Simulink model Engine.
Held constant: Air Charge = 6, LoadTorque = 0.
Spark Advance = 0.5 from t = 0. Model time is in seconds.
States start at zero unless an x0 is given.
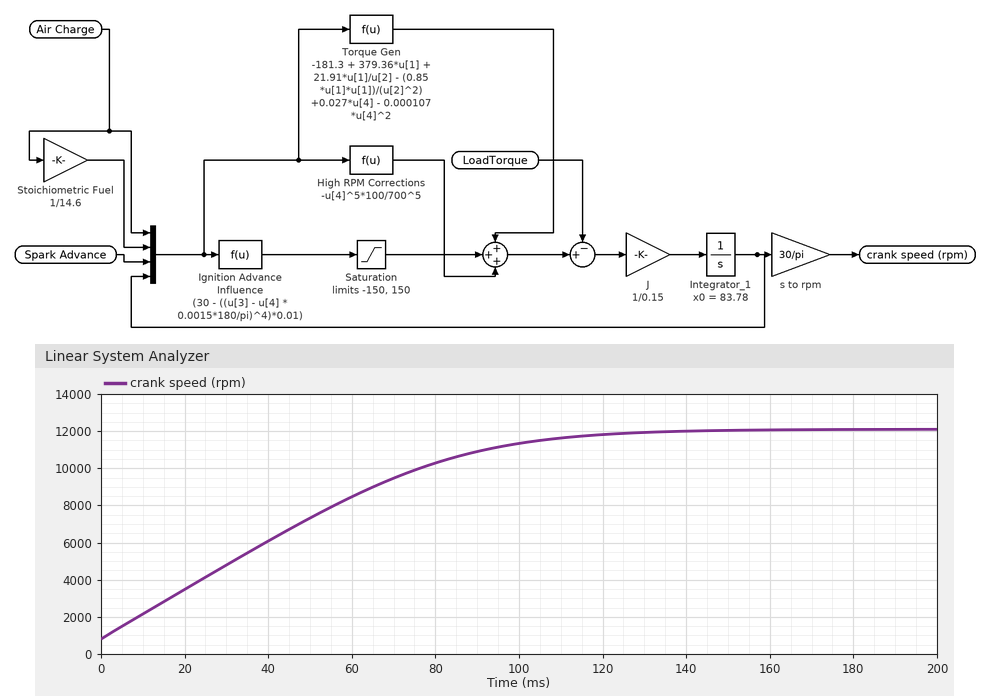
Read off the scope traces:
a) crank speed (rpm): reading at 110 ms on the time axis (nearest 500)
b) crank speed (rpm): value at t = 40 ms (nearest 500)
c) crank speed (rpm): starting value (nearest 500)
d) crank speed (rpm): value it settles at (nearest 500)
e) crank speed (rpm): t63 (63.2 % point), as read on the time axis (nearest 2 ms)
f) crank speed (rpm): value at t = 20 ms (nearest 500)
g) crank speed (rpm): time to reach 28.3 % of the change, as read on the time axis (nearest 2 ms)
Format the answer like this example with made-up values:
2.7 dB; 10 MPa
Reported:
11500; 6000; 1000; 12000; 56 ms; 3500; 24 ms
